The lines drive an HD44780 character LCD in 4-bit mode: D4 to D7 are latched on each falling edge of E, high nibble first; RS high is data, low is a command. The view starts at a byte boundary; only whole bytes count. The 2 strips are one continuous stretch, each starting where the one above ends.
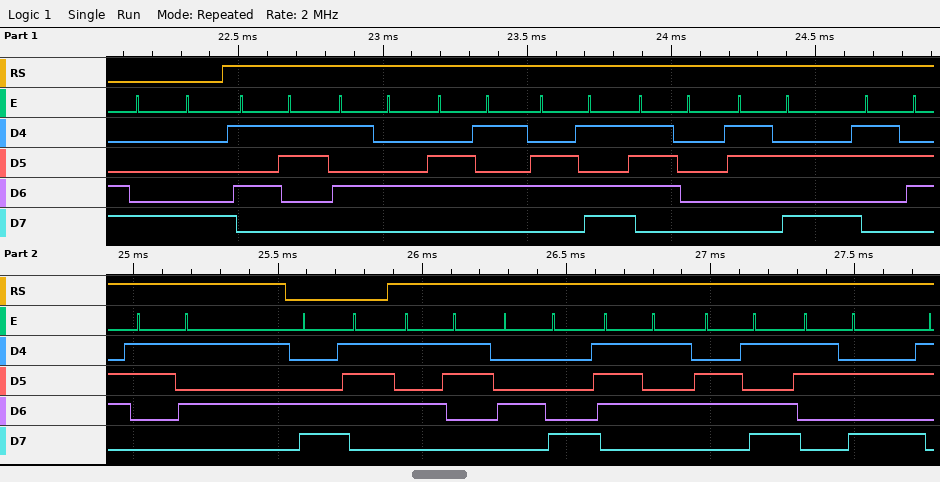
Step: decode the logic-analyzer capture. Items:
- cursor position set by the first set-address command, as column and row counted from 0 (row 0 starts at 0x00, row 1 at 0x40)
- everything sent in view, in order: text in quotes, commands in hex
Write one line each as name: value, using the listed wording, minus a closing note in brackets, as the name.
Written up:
cursor position set by the first set-address command, as column and row counted from 0: column 8, row 0
everything sent in view, in order: text in quotes, commands in hex: 0x88 "STemp:65" 0xC7 "SHum:"
